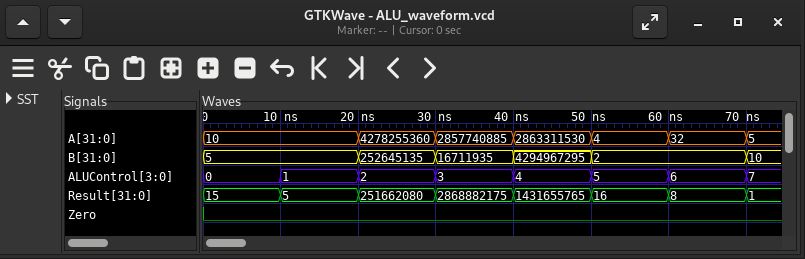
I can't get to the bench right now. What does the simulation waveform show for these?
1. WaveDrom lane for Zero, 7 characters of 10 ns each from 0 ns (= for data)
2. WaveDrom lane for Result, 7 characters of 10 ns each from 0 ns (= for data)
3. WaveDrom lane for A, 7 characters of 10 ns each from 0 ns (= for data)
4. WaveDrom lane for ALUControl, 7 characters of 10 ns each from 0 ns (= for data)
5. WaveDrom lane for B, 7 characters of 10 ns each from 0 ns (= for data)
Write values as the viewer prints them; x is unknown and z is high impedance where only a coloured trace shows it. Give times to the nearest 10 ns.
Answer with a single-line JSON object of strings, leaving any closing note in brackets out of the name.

{"WaveDrom lane for Zero, 7 characters of 10 ns each from 0 ns": "{name: 'Zero', wave: '0......'}", "WaveDrom lane for Result, 7 characters of 10 ns each from 0 ns": "{name: 'Result', wave: '=======', data: '15 5 251662080 2868882175 1431655765 16 8'}", "WaveDrom lane for A, 7 characters of 10 ns each from 0 ns": "{name: 'A', wave: '=.=====', data: '10 4278255360 2857740885 2863311530 4 32'}", "WaveDrom lane for ALUControl, 7 characters of 10 ns each from 0 ns": "{name: 'ALUControl', wave: '=======', data: '0 1 2 3 4 5 6'}", "WaveDrom lane for B, 7 characters of 10 ns each from 0 ns": "{name: 'B', wave: '=.====.', data: '5 252645135 16711935 4294967295 2'}"}
